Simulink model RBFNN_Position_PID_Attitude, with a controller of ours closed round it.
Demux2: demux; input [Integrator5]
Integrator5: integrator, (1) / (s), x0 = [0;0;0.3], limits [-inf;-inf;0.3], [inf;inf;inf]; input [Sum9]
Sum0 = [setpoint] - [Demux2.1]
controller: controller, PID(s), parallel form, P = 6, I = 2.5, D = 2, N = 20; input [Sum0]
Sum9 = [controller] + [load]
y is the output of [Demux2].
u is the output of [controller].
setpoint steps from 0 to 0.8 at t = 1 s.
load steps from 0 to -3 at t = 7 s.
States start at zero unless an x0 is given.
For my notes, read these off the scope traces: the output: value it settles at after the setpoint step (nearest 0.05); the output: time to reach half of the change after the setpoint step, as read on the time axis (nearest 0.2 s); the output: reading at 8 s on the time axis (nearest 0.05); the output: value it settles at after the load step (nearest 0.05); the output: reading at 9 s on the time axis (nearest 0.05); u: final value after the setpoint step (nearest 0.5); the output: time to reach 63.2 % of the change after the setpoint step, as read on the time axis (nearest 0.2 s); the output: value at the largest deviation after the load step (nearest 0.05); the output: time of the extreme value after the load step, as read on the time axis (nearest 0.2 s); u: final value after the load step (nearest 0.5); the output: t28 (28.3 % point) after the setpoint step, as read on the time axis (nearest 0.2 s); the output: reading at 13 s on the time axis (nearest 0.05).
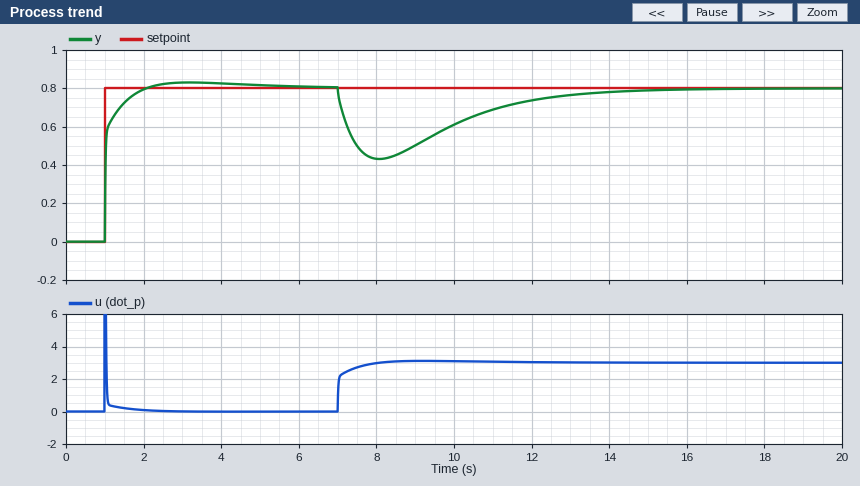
0.80
1.0 s
0.45
0.80
0.50
0.0
1.0 s
0.45
8.0 s
3.0
1.0 s
0.75
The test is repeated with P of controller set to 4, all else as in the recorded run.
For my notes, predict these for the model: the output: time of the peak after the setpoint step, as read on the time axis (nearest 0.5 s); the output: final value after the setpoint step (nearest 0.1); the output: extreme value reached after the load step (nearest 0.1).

3.5 s
0.8
0.3
